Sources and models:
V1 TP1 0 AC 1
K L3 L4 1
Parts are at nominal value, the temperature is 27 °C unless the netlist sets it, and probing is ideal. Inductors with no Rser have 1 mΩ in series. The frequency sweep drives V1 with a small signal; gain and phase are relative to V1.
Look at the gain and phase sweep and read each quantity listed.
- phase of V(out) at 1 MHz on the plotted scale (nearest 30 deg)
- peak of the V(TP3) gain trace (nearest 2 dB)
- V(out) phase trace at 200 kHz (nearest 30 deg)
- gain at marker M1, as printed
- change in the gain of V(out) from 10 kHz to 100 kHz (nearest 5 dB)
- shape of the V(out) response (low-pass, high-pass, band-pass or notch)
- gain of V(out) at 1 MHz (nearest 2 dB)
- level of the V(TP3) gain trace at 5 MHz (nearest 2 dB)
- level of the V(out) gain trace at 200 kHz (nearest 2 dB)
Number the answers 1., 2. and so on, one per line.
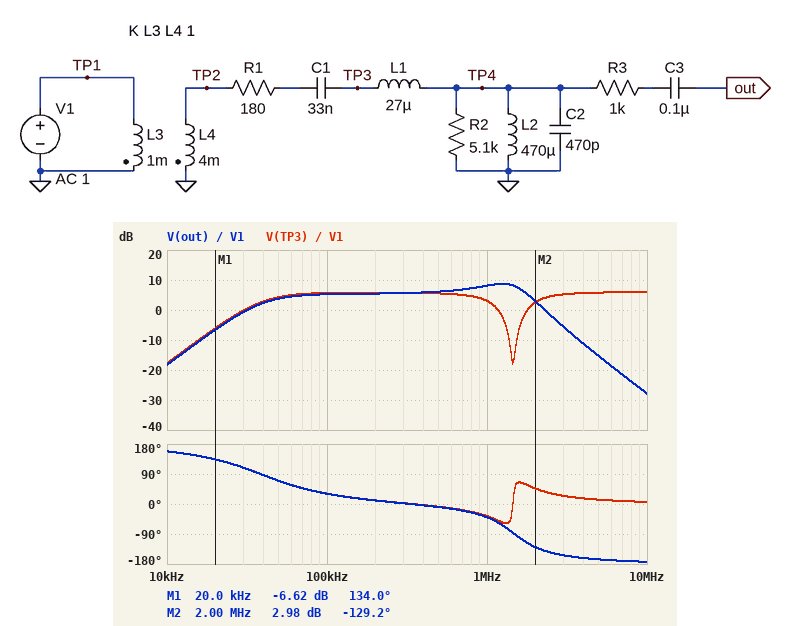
1. -30 deg
2. 6 dB
3. 0 deg
4. -6.62 dB
5. 25 dB
6. band-pass
7. 8 dB
8. 6 dB
9. 6 dB
